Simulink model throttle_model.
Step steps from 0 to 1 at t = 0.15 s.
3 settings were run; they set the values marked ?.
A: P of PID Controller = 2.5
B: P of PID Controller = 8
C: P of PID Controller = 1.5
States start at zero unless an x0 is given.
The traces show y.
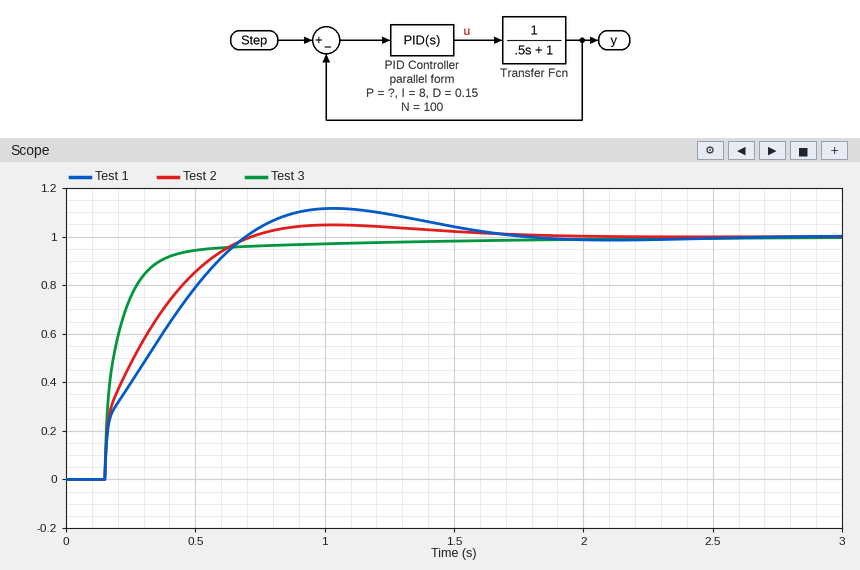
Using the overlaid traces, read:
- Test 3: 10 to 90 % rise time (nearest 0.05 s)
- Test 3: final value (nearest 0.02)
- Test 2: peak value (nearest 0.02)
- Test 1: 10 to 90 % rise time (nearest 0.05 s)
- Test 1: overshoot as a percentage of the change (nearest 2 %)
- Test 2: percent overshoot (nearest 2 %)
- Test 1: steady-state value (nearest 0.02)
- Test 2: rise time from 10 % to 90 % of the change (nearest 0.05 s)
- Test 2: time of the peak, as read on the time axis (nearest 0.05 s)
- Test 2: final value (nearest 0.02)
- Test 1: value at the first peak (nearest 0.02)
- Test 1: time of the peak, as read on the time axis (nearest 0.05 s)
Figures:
0.20 s
1.00
1.04
0.45 s
12 %
4 %
1.00
0.40 s
1.05 s
1.00
1.12
1.05 s
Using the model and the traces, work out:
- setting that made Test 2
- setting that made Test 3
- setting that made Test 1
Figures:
A
B
C
